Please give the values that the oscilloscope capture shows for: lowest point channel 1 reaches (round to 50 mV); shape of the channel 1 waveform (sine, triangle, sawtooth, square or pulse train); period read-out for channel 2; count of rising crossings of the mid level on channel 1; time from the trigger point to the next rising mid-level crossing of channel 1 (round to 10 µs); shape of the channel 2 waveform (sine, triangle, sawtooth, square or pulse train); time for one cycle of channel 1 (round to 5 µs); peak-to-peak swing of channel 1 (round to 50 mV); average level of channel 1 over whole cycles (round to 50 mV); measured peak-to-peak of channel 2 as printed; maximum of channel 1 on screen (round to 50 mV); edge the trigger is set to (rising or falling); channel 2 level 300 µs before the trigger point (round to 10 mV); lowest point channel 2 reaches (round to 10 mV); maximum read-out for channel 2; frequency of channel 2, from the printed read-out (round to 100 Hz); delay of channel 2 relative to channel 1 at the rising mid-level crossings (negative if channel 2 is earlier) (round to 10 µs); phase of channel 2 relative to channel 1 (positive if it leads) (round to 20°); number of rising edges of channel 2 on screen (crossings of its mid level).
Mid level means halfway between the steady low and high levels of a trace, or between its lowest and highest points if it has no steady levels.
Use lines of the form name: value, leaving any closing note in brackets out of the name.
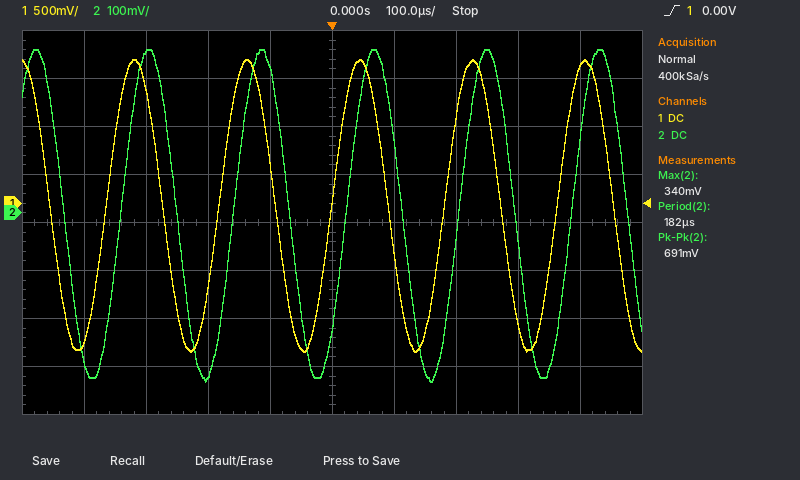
lowest point channel 1 reaches: -1.55 V
shape of the channel 1 waveform: sine
period read-out for channel 2: 182 µs
count of rising crossings of the mid level on channel 1: 5
time from the trigger point to the next rising mid-level crossing of channel 1: 180 µs
shape of the channel 2 waveform: sine
time for one cycle of channel 1: 180 µs
peak-to-peak swing of channel 1: 3.05 V
average level of channel 1 over whole cycles: 0 mV
measured peak-to-peak of channel 2 as printed: 691 mV
maximum of channel 1 on screen: 1.50 V
edge the trigger is set to: rising
channel 2 level 300 µs before the trigger point: 330 mV
lowest point channel 2 reaches: -350 mV
maximum read-out for channel 2: 340 mV
frequency of channel 2, from the printed read-out: 5.5 kHz
delay of channel 2 relative to channel 1 at the rising mid-level crossings (negative if channel 2 is earlier): +20 µs
phase of channel 2 relative to channel 1 (positive if it leads): -40°
number of rising edges of channel 2 on screen: 5
